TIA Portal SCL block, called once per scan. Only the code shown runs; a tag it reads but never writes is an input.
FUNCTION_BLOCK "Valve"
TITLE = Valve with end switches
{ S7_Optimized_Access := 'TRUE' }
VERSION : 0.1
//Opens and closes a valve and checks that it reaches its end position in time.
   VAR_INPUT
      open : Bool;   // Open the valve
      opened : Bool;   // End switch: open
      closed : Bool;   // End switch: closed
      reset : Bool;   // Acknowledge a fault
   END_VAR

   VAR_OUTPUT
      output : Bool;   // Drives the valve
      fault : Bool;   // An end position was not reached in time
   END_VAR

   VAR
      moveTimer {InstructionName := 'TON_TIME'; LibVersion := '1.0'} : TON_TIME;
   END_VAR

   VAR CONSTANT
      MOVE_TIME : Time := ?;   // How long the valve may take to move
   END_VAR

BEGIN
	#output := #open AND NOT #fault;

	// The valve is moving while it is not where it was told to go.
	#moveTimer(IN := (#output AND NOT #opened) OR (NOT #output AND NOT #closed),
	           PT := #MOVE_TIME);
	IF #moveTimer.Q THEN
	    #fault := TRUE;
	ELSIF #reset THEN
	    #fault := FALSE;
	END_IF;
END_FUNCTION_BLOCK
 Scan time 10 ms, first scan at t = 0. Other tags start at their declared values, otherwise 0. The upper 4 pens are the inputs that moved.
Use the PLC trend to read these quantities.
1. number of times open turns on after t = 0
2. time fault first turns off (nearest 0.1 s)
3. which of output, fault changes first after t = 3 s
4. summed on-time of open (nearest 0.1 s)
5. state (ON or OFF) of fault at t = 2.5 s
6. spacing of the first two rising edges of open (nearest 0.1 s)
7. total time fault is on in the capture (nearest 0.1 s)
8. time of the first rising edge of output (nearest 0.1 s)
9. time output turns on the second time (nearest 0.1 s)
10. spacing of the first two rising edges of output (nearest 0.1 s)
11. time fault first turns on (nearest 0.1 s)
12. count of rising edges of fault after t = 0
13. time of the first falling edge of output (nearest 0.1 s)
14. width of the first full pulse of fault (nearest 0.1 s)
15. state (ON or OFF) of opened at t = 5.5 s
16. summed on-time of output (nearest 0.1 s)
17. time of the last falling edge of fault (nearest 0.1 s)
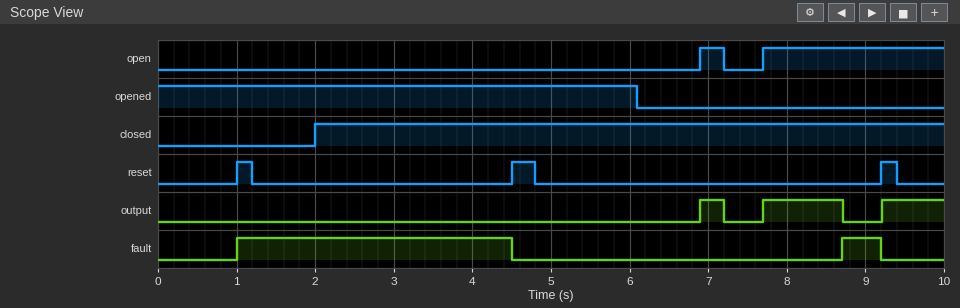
2
4.5 s
fault
2.6 s
ON
0.8 s
4.0 s
6.9 s
7.7 s
0.8 s
1.0 s
2
7.2 s
3.5 s
ON
2.1 s
9.2 s
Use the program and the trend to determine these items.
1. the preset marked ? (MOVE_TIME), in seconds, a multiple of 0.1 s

1.0 s
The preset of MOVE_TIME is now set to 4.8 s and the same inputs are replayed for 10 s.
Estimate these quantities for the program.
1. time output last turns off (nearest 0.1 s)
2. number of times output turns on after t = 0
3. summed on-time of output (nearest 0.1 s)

7.2 s
2
2.6 s
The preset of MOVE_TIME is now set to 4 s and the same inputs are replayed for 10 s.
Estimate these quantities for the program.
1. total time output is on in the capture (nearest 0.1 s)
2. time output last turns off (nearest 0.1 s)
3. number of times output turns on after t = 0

2.6 s
7.2 s
2
